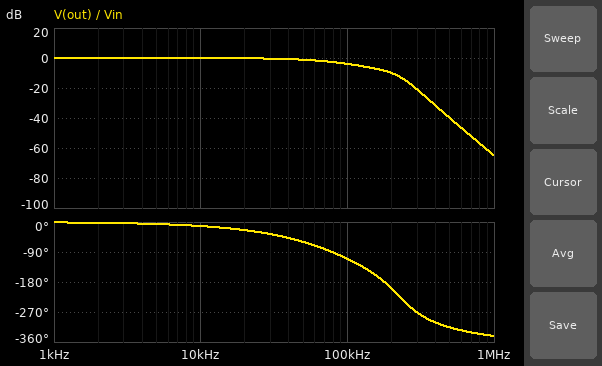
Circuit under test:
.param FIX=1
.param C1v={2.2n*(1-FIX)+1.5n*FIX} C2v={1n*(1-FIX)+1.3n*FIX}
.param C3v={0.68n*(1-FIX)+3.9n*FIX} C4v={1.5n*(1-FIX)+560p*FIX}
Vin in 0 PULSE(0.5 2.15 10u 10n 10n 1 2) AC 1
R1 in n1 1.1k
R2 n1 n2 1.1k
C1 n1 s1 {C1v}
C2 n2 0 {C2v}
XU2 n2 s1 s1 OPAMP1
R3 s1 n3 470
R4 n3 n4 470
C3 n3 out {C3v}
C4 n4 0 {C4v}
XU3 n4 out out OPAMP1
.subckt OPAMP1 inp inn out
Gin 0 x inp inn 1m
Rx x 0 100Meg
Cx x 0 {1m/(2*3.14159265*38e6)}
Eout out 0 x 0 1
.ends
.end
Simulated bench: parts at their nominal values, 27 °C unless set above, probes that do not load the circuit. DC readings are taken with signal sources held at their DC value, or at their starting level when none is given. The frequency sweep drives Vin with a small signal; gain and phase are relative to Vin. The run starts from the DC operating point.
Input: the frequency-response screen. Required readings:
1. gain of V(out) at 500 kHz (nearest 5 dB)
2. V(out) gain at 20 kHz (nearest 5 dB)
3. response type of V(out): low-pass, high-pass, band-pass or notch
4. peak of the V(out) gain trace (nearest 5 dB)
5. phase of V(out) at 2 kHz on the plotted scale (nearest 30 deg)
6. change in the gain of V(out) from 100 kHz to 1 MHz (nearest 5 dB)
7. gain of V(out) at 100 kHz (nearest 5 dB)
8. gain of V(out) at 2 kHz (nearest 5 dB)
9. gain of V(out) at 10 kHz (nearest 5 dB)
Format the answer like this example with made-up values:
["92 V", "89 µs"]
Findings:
["-40 dB", "0 dB", "low-pass", "0 dB", "0 deg", "-60 dB", "-5 dB", "0 dB", "0 dB"]
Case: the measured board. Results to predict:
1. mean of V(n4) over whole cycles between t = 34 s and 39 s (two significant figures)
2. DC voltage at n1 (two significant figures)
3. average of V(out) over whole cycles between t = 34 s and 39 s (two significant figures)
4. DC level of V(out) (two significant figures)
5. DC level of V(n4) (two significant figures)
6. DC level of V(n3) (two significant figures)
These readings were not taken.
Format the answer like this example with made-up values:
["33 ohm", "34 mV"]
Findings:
["1.3 V", "500 mV", "1.3 V", "500 mV", "500 mV", "500 mV"]
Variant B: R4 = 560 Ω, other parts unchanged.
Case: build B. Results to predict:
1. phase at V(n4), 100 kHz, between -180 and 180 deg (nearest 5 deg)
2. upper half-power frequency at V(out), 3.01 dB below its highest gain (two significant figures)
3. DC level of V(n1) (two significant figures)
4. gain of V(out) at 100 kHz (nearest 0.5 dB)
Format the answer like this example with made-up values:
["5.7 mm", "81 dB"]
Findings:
["-115 deg", "88 kHz", "500 mV", "-3.5 dB"]
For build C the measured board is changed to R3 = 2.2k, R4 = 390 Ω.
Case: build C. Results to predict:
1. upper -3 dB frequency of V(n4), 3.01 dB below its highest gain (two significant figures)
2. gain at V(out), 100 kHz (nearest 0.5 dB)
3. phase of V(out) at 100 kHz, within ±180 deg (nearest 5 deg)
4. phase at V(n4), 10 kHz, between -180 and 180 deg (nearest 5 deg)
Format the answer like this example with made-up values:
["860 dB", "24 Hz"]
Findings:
["86 kHz", "-4.5 dB", "-165 deg", "-15 deg"]
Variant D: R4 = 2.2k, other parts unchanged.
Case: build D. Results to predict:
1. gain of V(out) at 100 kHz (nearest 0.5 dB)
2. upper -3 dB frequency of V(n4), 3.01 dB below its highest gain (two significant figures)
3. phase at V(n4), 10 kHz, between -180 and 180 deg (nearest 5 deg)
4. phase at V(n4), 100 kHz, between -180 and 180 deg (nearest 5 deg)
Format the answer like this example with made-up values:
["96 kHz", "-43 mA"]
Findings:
["-4.5 dB", "88 kHz", "-15 deg", "-170 deg"]
